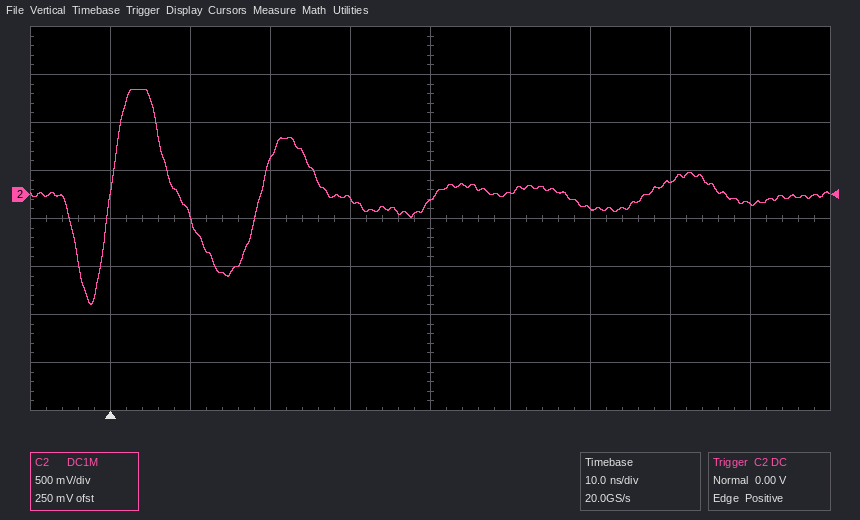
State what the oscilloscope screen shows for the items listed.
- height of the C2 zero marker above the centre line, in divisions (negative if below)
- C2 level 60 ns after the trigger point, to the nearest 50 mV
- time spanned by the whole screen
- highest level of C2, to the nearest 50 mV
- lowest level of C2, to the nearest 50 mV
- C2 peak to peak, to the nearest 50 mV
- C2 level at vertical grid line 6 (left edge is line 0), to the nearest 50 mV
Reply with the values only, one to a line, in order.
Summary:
+0.5 div
-150 mV
100 ns
1.10 V
-1.15 V
2.25 V
0 mV
